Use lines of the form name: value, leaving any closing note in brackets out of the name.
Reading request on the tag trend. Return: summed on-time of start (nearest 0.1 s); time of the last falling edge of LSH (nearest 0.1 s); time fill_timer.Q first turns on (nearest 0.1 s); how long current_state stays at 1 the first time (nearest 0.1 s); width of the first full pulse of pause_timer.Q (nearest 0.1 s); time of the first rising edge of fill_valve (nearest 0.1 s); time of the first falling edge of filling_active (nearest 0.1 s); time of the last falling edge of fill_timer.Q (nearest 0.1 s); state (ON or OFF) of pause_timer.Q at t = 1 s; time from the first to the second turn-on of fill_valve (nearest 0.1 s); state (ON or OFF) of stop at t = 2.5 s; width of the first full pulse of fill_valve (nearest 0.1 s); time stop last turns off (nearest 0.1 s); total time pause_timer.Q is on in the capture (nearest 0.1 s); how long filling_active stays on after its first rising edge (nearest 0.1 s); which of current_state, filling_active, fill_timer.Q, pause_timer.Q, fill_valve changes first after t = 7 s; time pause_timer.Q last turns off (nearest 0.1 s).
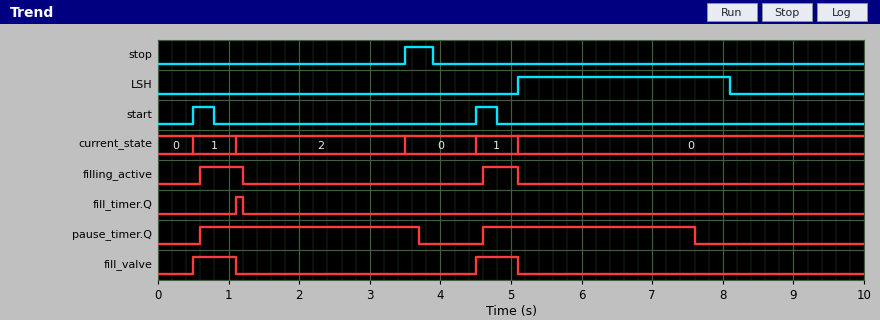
summed on-time of start: 0.6 s
time of the last falling edge of LSH: 8.1 s
time fill_timer.Q first turns on: 1.1 s
how long current_state stays at 1 the first time: 0.6 s
width of the first full pulse of pause_timer.Q: 3.1 s
time of the first rising edge of fill_valve: 0.5 s
time of the first falling edge of filling_active: 1.2 s
time of the last falling edge of fill_timer.Q: 1.2 s
state (ON or OFF) of pause_timer.Q at t = 1 s: ON
time from the first to the second turn-on of fill_valve: 4.0 s
state (ON or OFF) of stop at t = 2.5 s: OFF
width of the first full pulse of fill_valve: 0.6 s
time stop last turns off: 3.9 s
total time pause_timer.Q is on in the capture: 6.1 s
how long filling_active stays on after its first rising edge: 0.6 s
which of current_state, filling_active, fill_timer.Q, pause_timer.Q, fill_valve changes first after t = 7 s: pause_timer.Q
time pause_timer.Q last turns off: 7.6 s
